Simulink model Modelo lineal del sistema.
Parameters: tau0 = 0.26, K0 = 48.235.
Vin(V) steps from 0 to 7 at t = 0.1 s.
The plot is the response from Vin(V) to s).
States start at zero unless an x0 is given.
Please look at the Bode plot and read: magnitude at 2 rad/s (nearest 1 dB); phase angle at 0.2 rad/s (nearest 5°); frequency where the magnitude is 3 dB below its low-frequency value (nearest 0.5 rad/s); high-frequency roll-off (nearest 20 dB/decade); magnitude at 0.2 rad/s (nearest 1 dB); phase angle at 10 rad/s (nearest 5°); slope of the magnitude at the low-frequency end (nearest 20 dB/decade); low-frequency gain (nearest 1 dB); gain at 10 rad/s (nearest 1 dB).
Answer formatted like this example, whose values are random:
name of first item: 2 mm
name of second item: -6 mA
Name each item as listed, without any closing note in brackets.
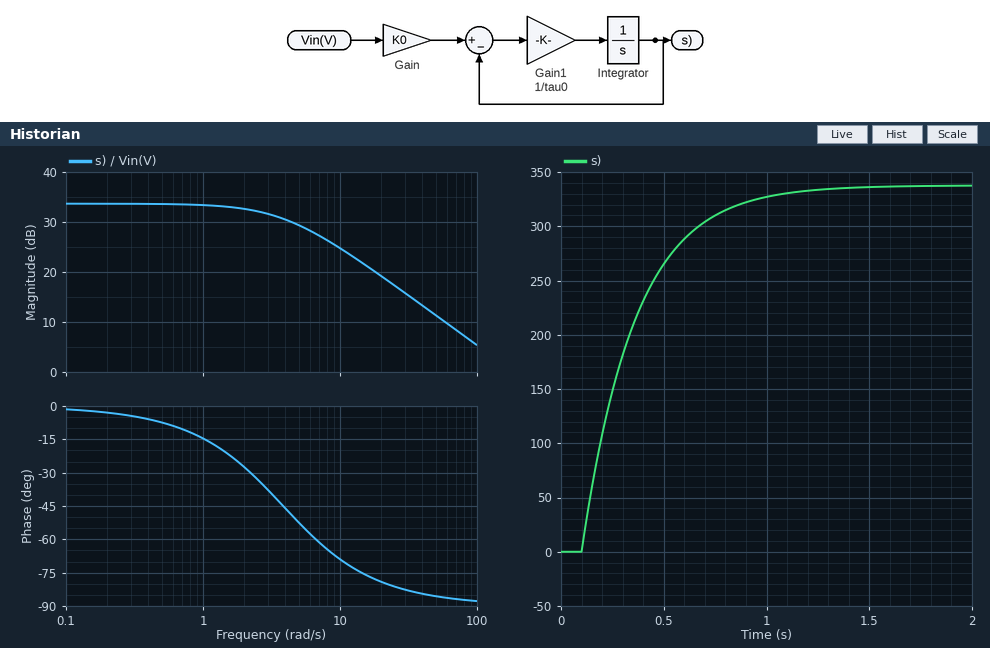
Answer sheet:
magnitude at 2 rad/s: 33 dB
phase angle at 0.2 rad/s: -5°
frequency where the magnitude is 3 dB below its low-frequency value: 4.0 rad/s
high-frequency roll-off: -20 dB/decade
magnitude at 0.2 rad/s: 34 dB
phase angle at 10 rad/s: -70°
slope of the magnitude at the low-frequency end: 0 dB/decade
low-frequency gain: 34 dB
gain at 10 rad/s: 25 dB
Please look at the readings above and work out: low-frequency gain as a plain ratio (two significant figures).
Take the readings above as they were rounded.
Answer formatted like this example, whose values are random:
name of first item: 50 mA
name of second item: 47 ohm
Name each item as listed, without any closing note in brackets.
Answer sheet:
low-frequency gain as a plain ratio: 50
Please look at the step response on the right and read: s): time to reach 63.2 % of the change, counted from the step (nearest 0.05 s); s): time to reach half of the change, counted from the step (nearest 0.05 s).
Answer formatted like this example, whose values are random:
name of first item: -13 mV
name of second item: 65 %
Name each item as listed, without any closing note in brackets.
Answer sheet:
s): time to reach 63.2 % of the change, counted from the step: 0.25 s
s): time to reach half of the change, counted from the step: 0.20 s
